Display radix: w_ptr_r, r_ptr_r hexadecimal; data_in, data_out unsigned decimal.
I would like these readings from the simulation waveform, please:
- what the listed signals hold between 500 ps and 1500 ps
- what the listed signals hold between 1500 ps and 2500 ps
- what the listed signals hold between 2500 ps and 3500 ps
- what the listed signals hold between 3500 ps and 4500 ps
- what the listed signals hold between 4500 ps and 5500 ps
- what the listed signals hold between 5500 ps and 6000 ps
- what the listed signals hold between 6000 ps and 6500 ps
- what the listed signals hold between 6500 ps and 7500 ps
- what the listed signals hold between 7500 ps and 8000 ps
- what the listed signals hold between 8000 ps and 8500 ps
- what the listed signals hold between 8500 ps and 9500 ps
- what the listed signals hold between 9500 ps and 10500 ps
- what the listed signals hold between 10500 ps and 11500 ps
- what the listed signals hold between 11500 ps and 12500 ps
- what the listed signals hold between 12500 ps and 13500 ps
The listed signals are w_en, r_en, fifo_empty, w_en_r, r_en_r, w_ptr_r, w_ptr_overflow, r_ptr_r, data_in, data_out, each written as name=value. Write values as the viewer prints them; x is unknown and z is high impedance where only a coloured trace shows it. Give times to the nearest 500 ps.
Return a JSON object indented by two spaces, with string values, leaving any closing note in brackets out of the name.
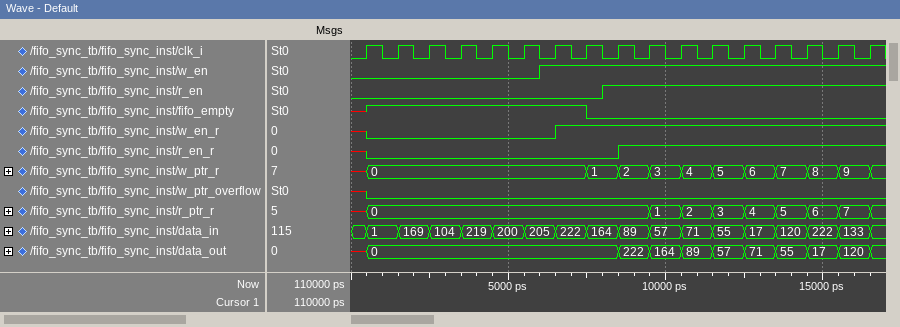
{
  "what the listed signals hold between 500 ps and 1500 ps": "w_en=0, r_en=0, fifo_empty=1, w_en_r=0, r_en_r=0, w_ptr_r=0, w_ptr_overflow=0, r_ptr_r=0, data_in=1, data_out=0",
  "what the listed signals hold between 1500 ps and 2500 ps": "w_en=0, r_en=0, fifo_empty=1, w_en_r=0, r_en_r=0, w_ptr_r=0, w_ptr_overflow=0, r_ptr_r=0, data_in=169, data_out=0",
  "what the listed signals hold between 2500 ps and 3500 ps": "w_en=0, r_en=0, fifo_empty=1, w_en_r=0, r_en_r=0, w_ptr_r=0, w_ptr_overflow=0, r_ptr_r=0, data_in=104, data_out=0",
  "what the listed signals hold between 3500 ps and 4500 ps": "w_en=0, r_en=0, fifo_empty=1, w_en_r=0, r_en_r=0, w_ptr_r=0, w_ptr_overflow=0, r_ptr_r=0, data_in=219, data_out=0",
  "what the listed signals hold between 4500 ps and 5500 ps": "w_en=0, r_en=0, fifo_empty=1, w_en_r=0, r_en_r=0, w_ptr_r=0, w_ptr_overflow=0, r_ptr_r=0, data_in=200, data_out=0",
  "what the listed signals hold between 5500 ps and 6000 ps": "w_en=0, r_en=0, fifo_empty=1, w_en_r=0, r_en_r=0, w_ptr_r=0, w_ptr_overflow=0, r_ptr_r=0, data_in=205, data_out=0",
  "what the listed signals hold between 6000 ps and 6500 ps": "w_en=1, r_en=0, fifo_empty=1, w_en_r=0, r_en_r=0, w_ptr_r=0, w_ptr_overflow=0, r_ptr_r=0, data_in=205, data_out=0",
  "what the listed signals hold between 6500 ps and 7500 ps": "w_en=1, r_en=0, fifo_empty=1, w_en_r=1, r_en_r=0, w_ptr_r=0, w_ptr_overflow=0, r_ptr_r=0, data_in=222, data_out=0",
  "what the listed signals hold between 7500 ps and 8000 ps": "w_en=1, r_en=0, fifo_empty=0, w_en_r=1, r_en_r=0, w_ptr_r=1, w_ptr_overflow=0, r_ptr_r=0, data_in=164, data_out=0",
  "what the listed signals hold between 8000 ps and 8500 ps": "w_en=1, r_en=1, fifo_empty=0, w_en_r=1, r_en_r=0, w_ptr_r=1, w_ptr_overflow=0, r_ptr_r=0, data_in=164, data_out=0",
  "what the listed signals hold between 8500 ps and 9500 ps": "w_en=1, r_en=1, fifo_empty=0, w_en_r=1, r_en_r=1, w_ptr_r=2, w_ptr_overflow=0, r_ptr_r=0, data_in=89, data_out=222",
  "what the listed signals hold between 9500 ps and 10500 ps": "w_en=1, r_en=1, fifo_empty=0, w_en_r=1, r_en_r=1, w_ptr_r=3, w_ptr_overflow=0, r_ptr_r=1, data_in=57, data_out=164",
  "what the listed signals hold between 10500 ps and 11500 ps": "w_en=1, r_en=1, fifo_empty=0, w_en_r=1, r_en_r=1, w_ptr_r=4, w_ptr_overflow=0, r_ptr_r=2, data_in=71, data_out=89",
  "what the listed signals hold between 11500 ps and 12500 ps": "w_en=1, r_en=1, fifo_empty=0, w_en_r=1, r_en_r=1, w_ptr_r=5, w_ptr_overflow=0, r_ptr_r=3, data_in=55, data_out=57",
  "what the listed signals hold between 12500 ps and 13500 ps": "w_en=1, r_en=1, fifo_empty=0, w_en_r=1, r_en_r=1, w_ptr_r=6, w_ptr_overflow=0, r_ptr_r=4, data_in=17, data_out=71"
}
